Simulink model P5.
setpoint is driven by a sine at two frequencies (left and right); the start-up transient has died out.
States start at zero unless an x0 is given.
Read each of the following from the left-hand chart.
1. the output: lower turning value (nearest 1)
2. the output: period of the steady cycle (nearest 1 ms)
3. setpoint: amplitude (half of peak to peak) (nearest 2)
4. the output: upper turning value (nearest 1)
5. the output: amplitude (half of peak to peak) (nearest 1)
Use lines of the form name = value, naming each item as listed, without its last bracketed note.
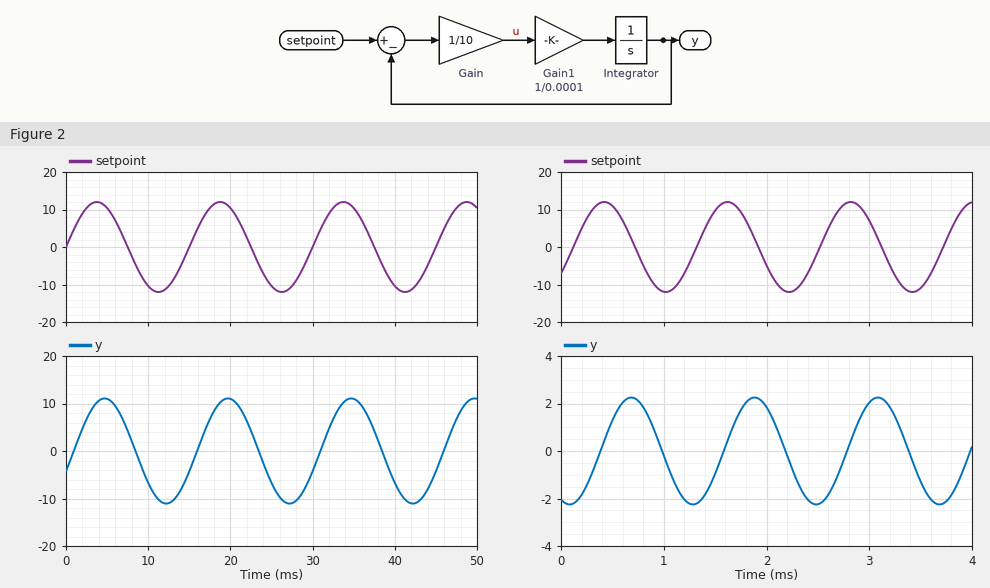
the output: lower turning value = -11
the output: period of the steady cycle = 15 ms
setpoint: amplitude (half of peak to peak) = 12
the output: upper turning value = 11
the output: amplitude (half of peak to peak) = 11
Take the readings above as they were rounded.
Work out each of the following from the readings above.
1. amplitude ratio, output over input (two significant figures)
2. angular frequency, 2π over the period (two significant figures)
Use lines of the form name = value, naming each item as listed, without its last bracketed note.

amplitude ratio, output over input = 0.92
angular frequency, 2π over the period = 0.42 rad/ms
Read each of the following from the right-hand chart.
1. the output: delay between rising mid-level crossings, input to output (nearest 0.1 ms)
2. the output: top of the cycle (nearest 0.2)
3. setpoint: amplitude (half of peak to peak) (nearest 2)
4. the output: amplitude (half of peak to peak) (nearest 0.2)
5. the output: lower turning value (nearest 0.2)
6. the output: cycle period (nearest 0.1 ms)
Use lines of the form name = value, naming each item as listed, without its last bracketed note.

the output: delay between rising mid-level crossings, input to output = 0.3 ms
the output: top of the cycle = 2.2
setpoint: amplitude (half of peak to peak) = 12
the output: amplitude (half of peak to peak) = 2.2
the output: lower turning value = -2.2
the output: cycle period = 1.2 ms
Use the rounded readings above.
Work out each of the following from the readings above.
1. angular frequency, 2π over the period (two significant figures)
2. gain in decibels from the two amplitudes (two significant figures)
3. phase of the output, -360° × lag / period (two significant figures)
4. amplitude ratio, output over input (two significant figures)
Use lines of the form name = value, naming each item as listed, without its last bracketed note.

angular frequency, 2π over the period = 5.2 rad/ms
gain in decibels from the two amplitudes = -15 dB
phase of the output, -360° × lag / period = -90°
amplitude ratio, output over input = 0.18
